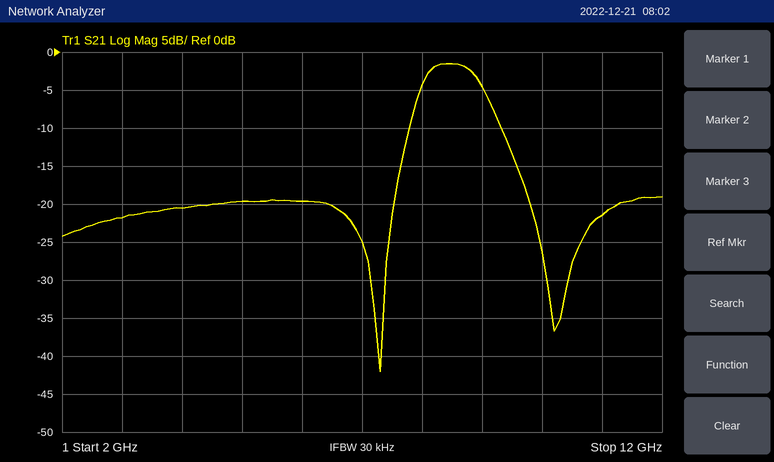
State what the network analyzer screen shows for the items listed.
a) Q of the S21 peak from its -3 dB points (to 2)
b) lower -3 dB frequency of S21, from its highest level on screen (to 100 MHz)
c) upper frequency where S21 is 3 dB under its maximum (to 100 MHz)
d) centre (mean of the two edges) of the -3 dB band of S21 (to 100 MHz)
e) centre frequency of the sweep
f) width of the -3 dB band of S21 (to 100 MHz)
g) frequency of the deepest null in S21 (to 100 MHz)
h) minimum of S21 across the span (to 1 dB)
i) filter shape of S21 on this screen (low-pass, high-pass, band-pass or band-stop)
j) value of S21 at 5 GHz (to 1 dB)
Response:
8
8.0 GHz
9.0 GHz
8.5 GHz
7 GHz
1.0 GHz
7.3 GHz
-42 dB
band-pass
-20 dB
